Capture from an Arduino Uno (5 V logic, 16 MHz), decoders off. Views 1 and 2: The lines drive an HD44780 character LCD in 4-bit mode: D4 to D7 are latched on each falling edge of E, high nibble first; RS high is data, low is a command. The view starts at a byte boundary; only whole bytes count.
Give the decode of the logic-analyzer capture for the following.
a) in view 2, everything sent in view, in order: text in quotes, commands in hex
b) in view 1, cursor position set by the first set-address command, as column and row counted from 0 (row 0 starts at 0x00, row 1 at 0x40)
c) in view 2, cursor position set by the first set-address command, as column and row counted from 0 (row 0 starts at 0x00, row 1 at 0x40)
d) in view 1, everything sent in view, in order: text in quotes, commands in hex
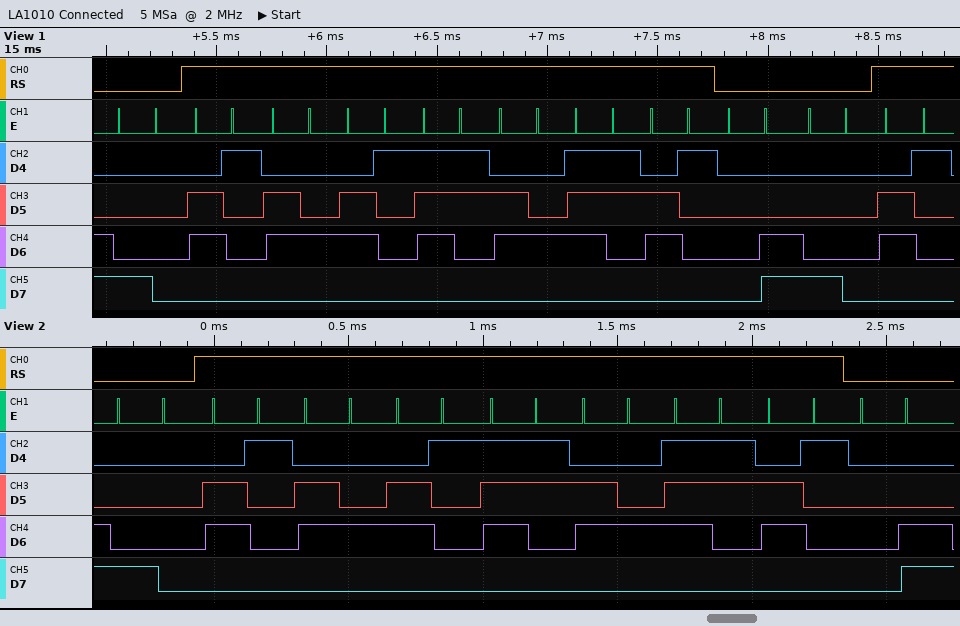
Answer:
0x80 "adasdsa" 0x0C
column 0, row 0
column 0, row 0
0x80 "adasdsa" 0x0C 0x80 "a"
